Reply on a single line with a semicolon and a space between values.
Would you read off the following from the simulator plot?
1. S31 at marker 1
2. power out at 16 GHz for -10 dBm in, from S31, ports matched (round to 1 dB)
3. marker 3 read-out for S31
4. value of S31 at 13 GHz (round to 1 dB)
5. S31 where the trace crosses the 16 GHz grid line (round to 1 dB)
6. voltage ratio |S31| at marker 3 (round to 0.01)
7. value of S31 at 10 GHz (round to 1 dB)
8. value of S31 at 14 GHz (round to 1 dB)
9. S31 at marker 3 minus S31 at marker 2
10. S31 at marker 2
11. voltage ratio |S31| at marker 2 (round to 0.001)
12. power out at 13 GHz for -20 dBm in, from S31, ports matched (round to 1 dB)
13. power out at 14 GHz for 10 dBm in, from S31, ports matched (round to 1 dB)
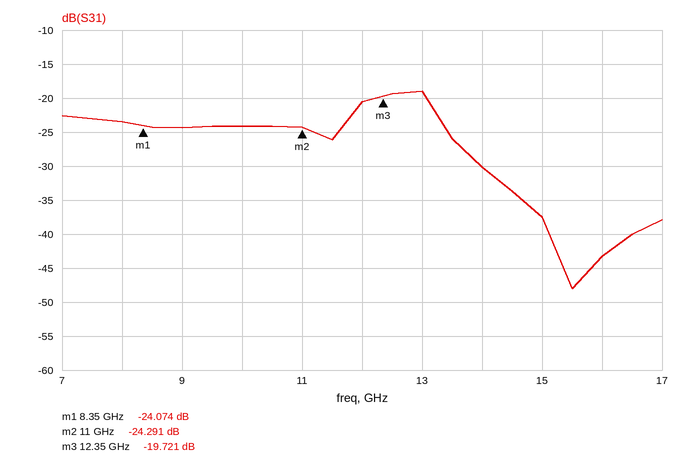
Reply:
-24.074 dB; -53 dBm; -19.721 dB; -19 dB; -43 dB; 0.10; -24 dB; -30 dB; 4.570 dB; -24.291 dB; 0.061; -39 dBm; -20 dBm
